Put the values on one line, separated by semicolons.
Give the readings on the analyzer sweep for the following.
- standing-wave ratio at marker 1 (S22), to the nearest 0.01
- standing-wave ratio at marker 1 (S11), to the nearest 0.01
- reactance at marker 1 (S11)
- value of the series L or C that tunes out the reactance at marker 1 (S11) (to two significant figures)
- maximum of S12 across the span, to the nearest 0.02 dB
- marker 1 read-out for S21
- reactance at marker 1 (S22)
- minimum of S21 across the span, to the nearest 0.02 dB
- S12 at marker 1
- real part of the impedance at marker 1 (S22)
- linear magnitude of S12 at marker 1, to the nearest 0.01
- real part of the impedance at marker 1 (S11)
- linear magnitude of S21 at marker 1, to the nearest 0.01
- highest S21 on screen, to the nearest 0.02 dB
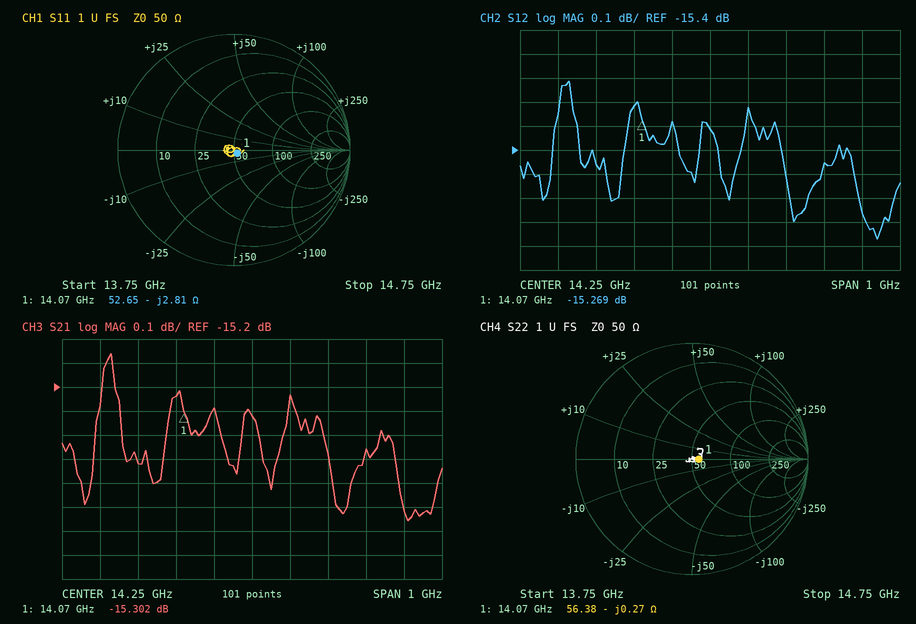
1.13; 1.08; -2.81 Ω; 32 pH; -15.12 dB; -15.302 dB; -0.27 Ω; -15.76 dB; -15.269 dB; 56.38 Ω; 0.17; 52.65 Ω; 0.17; -15.06 dB
